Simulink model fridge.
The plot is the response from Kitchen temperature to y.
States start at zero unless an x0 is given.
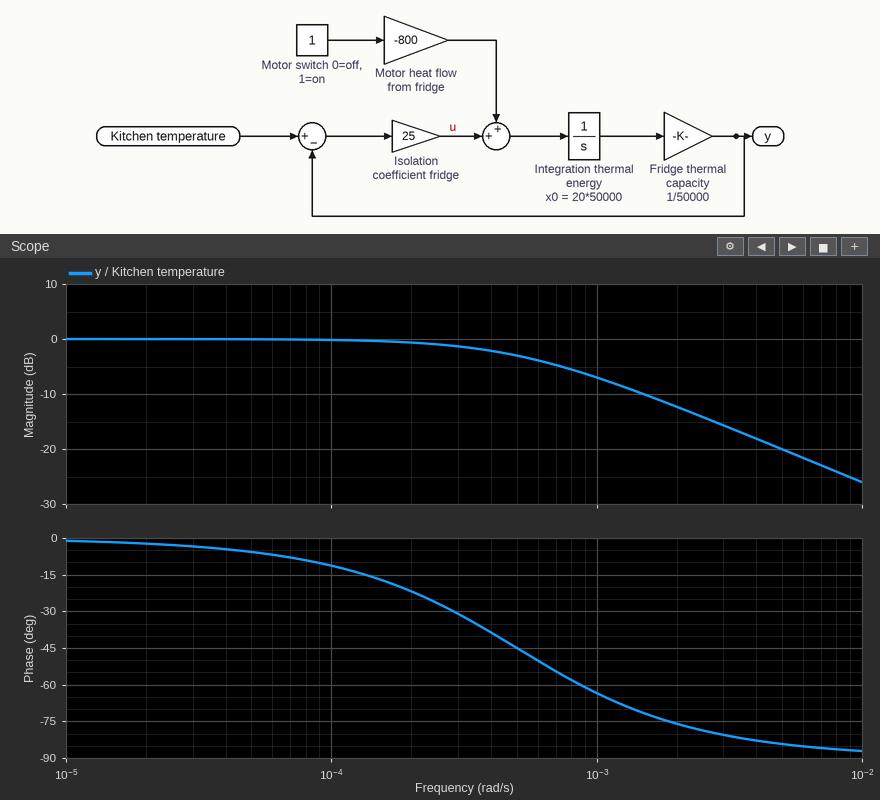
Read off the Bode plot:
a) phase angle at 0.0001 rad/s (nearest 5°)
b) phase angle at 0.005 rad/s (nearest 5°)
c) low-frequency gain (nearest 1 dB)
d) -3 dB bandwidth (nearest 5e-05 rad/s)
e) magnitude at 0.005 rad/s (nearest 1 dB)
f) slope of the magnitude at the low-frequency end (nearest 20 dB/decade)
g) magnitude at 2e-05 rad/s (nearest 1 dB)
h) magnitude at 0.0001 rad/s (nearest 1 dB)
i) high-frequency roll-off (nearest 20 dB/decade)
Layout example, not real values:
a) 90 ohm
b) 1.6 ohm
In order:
a) -10°
b) -85°
c) 0 dB
d) 0.00050 rad/s
e) -20 dB
f) 0 dB/decade
g) 0 dB
h) 0 dB
i) -20 dB/decade
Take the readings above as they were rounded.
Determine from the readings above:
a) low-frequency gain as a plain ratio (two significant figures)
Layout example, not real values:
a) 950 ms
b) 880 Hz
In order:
a) 1.0
